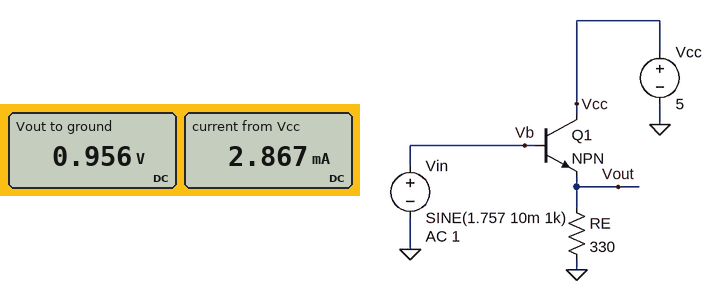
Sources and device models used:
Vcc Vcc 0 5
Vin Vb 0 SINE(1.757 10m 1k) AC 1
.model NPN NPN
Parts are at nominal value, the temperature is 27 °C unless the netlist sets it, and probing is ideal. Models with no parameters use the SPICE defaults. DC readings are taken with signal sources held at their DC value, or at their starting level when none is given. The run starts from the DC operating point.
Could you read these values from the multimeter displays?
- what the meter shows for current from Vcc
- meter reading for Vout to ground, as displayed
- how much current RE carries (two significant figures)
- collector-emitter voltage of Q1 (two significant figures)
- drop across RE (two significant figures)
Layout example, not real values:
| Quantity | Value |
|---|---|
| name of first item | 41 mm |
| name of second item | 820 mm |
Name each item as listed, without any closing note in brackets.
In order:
| Quantity | Value |
|---|---|
| what the meter shows for current from Vcc | 2.867 mA |
| meter reading for Vout to ground, as displayed | 0.956 V |
| how much current RE carries | 2.9 mA |
| collector-emitter voltage of Q1 | 4.0 V |
| drop across RE | 960 mV |
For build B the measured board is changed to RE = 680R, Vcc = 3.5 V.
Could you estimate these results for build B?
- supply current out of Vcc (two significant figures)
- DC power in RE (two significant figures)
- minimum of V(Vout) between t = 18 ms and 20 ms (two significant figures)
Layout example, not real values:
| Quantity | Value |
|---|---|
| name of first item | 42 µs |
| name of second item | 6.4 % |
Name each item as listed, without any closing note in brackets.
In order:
| Quantity | Value |
|---|---|
| supply current out of Vcc | 1.4 mA |
| DC power in RE | 1.4 mW |
| minimum of V(Vout) between t = 18 ms and 20 ms | 960 mV |
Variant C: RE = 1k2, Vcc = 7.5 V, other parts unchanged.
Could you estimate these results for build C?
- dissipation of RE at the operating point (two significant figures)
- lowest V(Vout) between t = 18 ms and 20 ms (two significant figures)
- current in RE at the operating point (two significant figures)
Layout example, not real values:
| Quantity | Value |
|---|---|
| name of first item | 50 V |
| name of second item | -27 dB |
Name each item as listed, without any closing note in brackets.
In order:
| Quantity | Value |
|---|---|
| dissipation of RE at the operating point | 810 µW |
| lowest V(Vout) between t = 18 ms and 20 ms | 980 mV |
| current in RE at the operating point | 820 µA |
